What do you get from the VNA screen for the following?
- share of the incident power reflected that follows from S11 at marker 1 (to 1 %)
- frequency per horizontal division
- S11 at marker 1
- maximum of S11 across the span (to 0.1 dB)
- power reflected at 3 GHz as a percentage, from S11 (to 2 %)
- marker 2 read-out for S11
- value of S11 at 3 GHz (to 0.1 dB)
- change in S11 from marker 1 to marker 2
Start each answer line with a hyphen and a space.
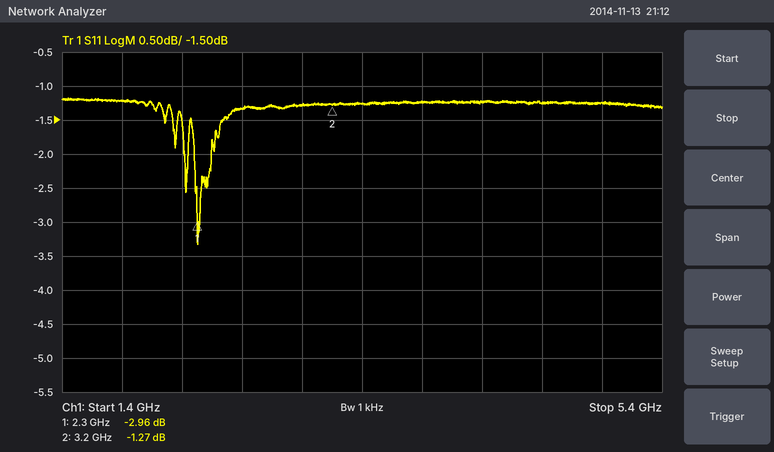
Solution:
- 51 %
- 400 MHz
- -2.96 dB
- -1.2 dB
- 74 %
- -1.27 dB
- -1.3 dB
- 1.69 dB
